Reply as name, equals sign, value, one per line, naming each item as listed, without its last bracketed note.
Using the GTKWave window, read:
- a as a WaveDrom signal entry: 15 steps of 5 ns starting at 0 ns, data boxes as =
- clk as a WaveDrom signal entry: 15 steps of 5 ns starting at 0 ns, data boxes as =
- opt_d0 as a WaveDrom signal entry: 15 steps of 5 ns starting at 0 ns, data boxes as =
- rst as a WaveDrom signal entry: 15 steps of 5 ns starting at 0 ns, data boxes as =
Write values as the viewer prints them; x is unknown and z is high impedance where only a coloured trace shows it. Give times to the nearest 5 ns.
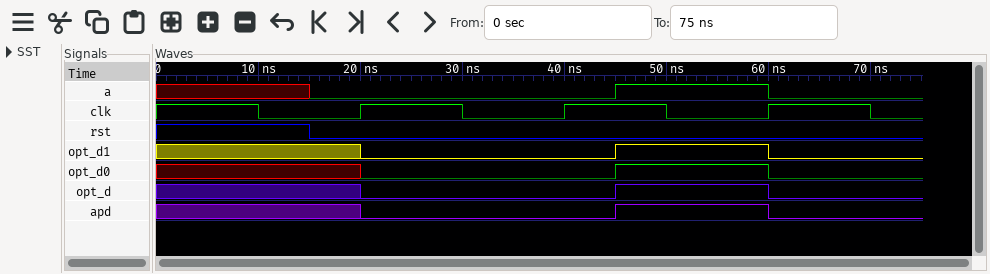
a as a WaveDrom signal entry: 15 steps of 5 ns starting at 0 ns, data boxes as = = {name: 'a', wave: 'x..0.....1..0..'}
clk as a WaveDrom signal entry: 15 steps of 5 ns starting at 0 ns, data boxes as = = {name: 'clk', wave: '1.0.1.0.1.0.1.0'}
opt_d0 as a WaveDrom signal entry: 15 steps of 5 ns starting at 0 ns, data boxes as = = {name: 'opt_d0', wave: 'x...0....1..0..'}
rst as a WaveDrom signal entry: 15 steps of 5 ns starting at 0 ns, data boxes as = = {name: 'rst', wave: '1..0...........'}
